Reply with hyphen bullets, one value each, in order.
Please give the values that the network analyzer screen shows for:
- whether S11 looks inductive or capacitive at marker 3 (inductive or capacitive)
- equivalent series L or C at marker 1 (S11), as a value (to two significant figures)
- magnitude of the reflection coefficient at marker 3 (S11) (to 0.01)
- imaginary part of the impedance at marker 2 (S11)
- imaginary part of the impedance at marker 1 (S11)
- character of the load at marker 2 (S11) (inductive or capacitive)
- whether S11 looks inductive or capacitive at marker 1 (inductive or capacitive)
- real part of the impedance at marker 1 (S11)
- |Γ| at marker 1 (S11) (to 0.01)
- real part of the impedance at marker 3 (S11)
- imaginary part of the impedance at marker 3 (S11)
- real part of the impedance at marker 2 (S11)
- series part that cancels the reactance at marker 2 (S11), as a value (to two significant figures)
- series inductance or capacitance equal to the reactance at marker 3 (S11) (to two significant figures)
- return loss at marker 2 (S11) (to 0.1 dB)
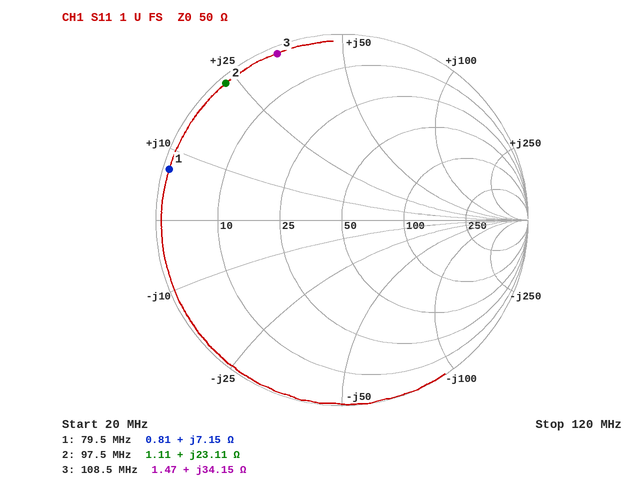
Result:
- inductive
- 14 nH
- 0.96
- +23.11 Ω
- +7.15 Ω
- inductive
- inductive
- 0.81 Ω
- 0.97
- 1.47 Ω
- +34.15 Ω
- 1.11 Ω
- 71 pF
- 50 nH
- 0.3 dB
